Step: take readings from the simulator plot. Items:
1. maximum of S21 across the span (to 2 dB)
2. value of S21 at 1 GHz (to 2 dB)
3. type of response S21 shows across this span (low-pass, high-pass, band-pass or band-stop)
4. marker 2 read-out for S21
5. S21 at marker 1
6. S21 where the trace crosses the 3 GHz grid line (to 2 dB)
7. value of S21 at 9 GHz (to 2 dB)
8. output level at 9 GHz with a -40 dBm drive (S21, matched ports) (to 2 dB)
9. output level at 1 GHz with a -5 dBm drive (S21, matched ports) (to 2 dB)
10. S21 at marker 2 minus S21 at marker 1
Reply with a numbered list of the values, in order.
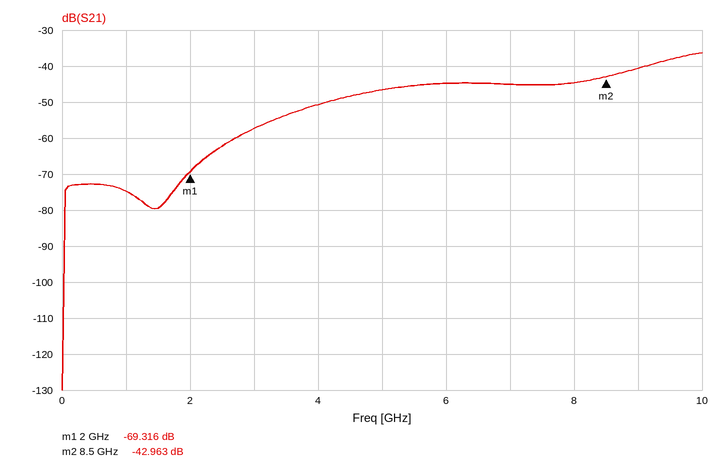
1. -36 dB
2. -74 dB
3. high-pass
4. -42.963 dB
5. -69.316 dB
6. -58 dB
7. -40 dB
8. -80 dBm
9. -80 dBm
10. 26.353 dB
